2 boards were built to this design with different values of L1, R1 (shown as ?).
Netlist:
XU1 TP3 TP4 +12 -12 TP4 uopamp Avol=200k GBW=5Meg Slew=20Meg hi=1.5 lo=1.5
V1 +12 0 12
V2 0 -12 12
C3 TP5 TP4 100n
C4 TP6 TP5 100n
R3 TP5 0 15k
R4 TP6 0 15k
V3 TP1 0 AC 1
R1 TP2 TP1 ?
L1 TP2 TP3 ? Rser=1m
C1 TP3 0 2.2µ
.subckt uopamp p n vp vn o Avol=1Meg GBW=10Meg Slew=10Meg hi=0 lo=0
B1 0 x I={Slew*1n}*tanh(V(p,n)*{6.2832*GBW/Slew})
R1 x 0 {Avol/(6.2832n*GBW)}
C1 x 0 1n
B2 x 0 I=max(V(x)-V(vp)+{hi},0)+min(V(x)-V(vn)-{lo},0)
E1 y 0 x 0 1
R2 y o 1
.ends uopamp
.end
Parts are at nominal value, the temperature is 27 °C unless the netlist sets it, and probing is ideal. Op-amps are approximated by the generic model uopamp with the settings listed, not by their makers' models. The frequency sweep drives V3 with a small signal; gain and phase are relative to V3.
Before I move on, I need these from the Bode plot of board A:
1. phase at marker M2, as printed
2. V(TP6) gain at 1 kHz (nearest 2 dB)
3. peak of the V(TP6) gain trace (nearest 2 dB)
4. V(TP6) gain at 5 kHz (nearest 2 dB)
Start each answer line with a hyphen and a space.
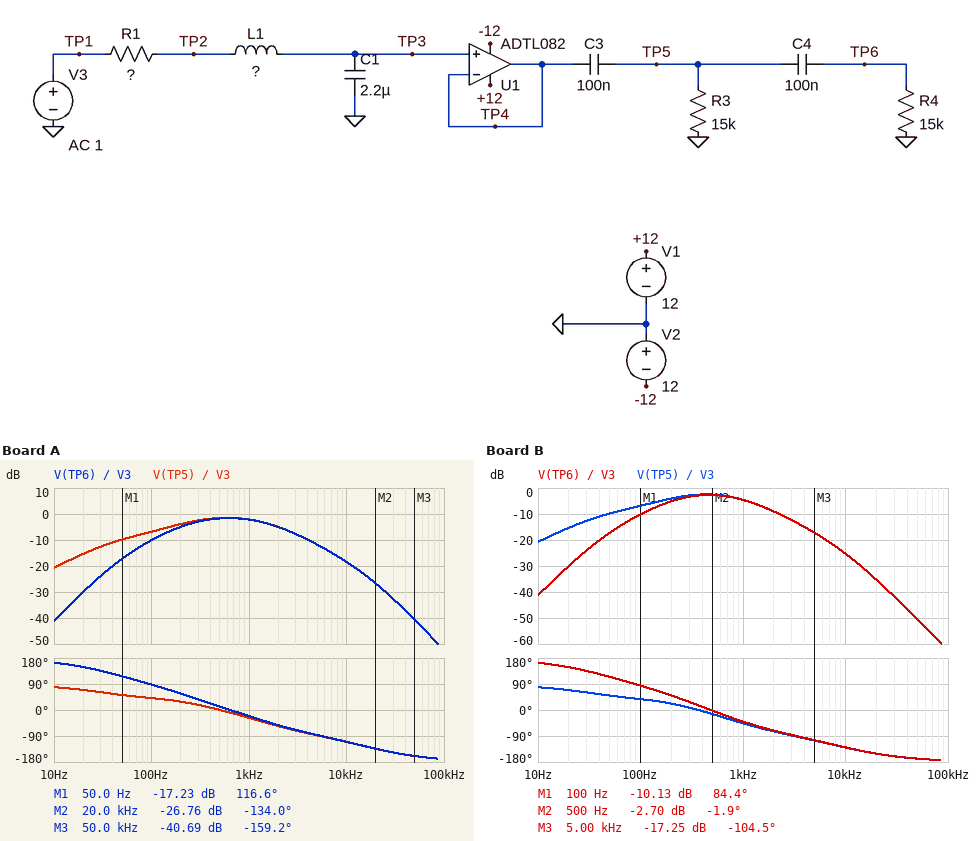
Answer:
- -134.0 deg
- -2 dB
- -2 dB
- -12 dB
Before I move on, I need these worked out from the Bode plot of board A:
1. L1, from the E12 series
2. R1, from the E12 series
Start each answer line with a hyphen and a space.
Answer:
- 470 µH
- 56 Ω
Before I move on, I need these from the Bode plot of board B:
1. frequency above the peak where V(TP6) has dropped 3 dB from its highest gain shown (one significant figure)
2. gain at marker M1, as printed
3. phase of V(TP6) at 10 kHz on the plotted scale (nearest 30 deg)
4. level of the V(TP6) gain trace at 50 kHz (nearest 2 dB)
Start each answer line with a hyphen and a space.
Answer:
- 1 kHz
- -10.13 dB
- -120 deg
- -50 dB
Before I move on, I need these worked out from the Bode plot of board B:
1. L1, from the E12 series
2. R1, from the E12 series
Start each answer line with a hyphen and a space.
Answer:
- 1.5 mH
- 100 Ω
